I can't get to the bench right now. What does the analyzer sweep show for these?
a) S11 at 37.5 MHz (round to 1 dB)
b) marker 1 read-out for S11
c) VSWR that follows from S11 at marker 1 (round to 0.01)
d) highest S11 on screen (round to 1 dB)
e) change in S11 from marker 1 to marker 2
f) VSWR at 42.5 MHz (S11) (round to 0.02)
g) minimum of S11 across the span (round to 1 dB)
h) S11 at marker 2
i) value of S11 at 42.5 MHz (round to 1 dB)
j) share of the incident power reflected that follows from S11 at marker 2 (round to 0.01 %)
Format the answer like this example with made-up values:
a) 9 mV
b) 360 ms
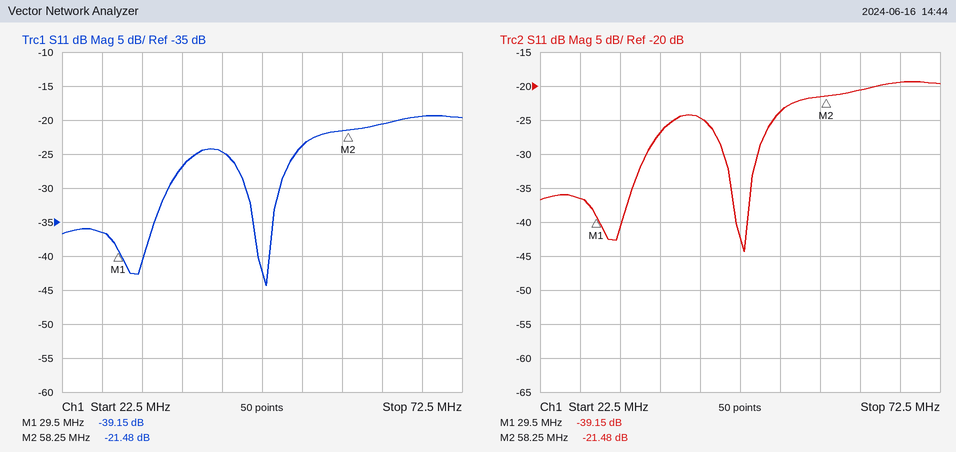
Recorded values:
a) -27 dB
b) -39.15 dB
c) 1.02
d) -19 dB
e) 17.67 dB
f) 1.12
g) -44 dB
h) -21.48 dB
i) -25 dB
j) 0.71 %
